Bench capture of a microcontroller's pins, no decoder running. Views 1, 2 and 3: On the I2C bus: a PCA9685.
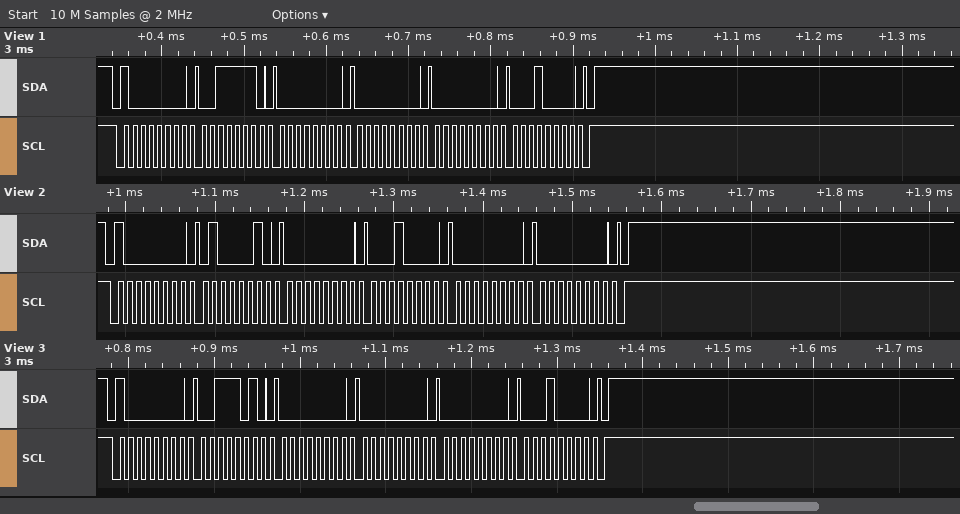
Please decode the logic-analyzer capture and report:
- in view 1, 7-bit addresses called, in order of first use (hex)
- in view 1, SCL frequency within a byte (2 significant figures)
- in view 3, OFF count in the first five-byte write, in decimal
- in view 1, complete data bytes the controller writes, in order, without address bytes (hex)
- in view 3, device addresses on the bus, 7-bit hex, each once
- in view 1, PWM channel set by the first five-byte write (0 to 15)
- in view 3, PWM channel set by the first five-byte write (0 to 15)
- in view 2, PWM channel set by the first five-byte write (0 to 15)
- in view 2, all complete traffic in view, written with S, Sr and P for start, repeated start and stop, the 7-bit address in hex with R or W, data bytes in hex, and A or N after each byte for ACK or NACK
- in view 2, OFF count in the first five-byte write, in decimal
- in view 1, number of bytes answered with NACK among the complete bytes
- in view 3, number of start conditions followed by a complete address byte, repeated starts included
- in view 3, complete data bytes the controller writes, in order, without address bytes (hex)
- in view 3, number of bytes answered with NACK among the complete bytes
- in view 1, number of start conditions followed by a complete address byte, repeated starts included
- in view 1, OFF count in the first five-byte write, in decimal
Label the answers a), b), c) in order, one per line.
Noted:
a) 0x40
b) 100 kHz
c) 4096
d) 3E 00 00 00 10
e) 0x40
f) 14
g) 13
h) 15
i) S 40W A 42 A 00 A 10 A 00 A 00 A P
j) 0
k) 0
l) 1
m) 3A 00 00 00 10
n) 0
o) 1
p) 4096
